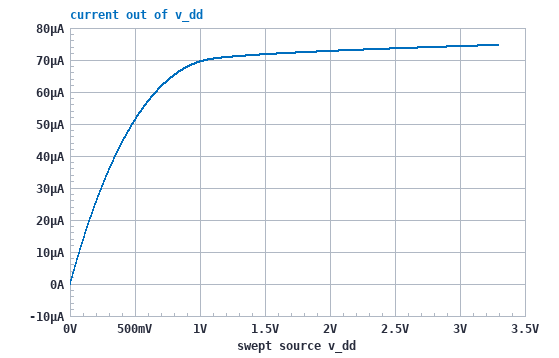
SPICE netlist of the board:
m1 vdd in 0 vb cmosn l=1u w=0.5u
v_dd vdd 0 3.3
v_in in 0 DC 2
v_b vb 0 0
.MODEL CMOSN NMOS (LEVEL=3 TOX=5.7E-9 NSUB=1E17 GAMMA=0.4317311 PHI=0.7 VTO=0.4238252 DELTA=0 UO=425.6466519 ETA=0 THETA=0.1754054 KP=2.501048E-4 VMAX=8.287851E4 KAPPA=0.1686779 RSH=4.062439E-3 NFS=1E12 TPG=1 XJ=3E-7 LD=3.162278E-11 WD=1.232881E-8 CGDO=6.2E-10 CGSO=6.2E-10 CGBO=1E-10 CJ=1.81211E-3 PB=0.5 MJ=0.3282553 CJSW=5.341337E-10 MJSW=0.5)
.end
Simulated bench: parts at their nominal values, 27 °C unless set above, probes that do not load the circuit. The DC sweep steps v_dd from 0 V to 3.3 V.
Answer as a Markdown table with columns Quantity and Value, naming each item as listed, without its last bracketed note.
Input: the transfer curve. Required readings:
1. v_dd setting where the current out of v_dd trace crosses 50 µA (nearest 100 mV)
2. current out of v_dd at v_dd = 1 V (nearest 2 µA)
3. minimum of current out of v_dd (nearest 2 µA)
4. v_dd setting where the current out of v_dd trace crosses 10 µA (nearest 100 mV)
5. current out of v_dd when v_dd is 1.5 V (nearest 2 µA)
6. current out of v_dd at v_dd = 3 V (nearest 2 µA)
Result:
| Quantity | Value |
|---|---|
| v_dd setting where the current out of v_dd trace crosses 50 µA | 500 mV |
| current out of v_dd at v_dd = 1 V | 70 µA |
| minimum of current out of v_dd | 0 A |
| v_dd setting where the current out of v_dd trace crosses 10 µA | 100 mV |
| current out of v_dd when v_dd is 1.5 V | 72 µA |
| current out of v_dd at v_dd = 3 V | 74 µA |
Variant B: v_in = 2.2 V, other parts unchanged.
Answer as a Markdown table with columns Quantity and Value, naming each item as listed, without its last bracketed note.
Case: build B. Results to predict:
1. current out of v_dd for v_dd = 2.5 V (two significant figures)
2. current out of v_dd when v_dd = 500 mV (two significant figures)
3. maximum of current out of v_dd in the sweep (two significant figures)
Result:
| Quantity | Value |
|---|---|
| current out of v_dd for v_dd = 2.5 V | 88 µA |
| current out of v_dd when v_dd = 500 mV | 58 µA |
| maximum of current out of v_dd in the sweep | 89 µA |
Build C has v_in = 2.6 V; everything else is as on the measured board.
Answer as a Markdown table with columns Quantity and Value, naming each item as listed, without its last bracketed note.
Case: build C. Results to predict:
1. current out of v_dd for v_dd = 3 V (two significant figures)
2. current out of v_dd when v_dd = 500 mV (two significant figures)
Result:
| Quantity | Value |
|---|---|
| current out of v_dd for v_dd = 3 V | 120 µA |
| current out of v_dd when v_dd = 500 mV | 70 µA |
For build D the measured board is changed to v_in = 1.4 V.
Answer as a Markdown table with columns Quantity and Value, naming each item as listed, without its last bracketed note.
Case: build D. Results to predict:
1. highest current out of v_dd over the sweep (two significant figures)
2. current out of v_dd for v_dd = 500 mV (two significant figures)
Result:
| Quantity | Value |
|---|---|
| highest current out of v_dd over the sweep | 36 µA |
| current out of v_dd for v_dd = 500 mV | 30 µA |
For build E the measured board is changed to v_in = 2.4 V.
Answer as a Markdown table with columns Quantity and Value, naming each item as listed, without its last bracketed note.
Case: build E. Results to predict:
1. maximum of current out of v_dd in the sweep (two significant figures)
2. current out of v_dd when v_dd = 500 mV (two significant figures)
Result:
| Quantity | Value |
|---|---|
| maximum of current out of v_dd in the sweep | 100 µA |
| current out of v_dd when v_dd = 500 mV | 64 µA |
